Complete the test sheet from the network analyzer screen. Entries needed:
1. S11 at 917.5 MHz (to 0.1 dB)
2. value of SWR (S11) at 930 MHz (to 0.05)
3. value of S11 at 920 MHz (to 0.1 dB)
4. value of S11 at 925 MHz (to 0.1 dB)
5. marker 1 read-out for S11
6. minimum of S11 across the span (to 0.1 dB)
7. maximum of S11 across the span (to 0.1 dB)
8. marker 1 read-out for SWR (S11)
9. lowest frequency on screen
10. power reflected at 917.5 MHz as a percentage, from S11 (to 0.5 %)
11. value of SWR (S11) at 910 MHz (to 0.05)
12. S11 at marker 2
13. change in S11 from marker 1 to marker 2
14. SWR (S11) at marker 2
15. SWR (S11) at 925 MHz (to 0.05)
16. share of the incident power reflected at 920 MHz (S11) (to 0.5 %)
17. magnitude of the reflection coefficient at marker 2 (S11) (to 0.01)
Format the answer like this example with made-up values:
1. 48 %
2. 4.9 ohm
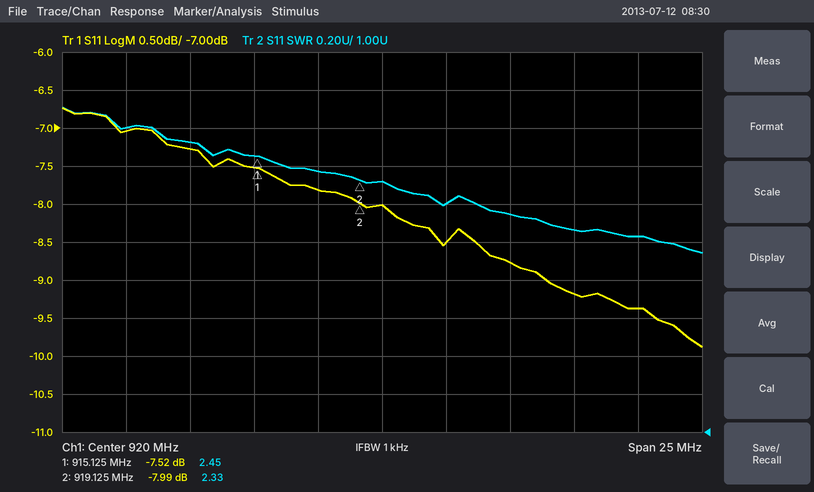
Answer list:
1. -7.8 dB
2. 2.05
3. -8.0 dB
4. -8.8 dB
5. -7.52 dB
6. -9.9 dB
7. -6.7 dB
8. 2.45
9. 907.5 MHz
10. 16.5 %
11. 2.60
12. -7.99 dB
13. -0.47 dB
14. 2.33
15. 2.15
16. 16.0 %
17. 0.40
